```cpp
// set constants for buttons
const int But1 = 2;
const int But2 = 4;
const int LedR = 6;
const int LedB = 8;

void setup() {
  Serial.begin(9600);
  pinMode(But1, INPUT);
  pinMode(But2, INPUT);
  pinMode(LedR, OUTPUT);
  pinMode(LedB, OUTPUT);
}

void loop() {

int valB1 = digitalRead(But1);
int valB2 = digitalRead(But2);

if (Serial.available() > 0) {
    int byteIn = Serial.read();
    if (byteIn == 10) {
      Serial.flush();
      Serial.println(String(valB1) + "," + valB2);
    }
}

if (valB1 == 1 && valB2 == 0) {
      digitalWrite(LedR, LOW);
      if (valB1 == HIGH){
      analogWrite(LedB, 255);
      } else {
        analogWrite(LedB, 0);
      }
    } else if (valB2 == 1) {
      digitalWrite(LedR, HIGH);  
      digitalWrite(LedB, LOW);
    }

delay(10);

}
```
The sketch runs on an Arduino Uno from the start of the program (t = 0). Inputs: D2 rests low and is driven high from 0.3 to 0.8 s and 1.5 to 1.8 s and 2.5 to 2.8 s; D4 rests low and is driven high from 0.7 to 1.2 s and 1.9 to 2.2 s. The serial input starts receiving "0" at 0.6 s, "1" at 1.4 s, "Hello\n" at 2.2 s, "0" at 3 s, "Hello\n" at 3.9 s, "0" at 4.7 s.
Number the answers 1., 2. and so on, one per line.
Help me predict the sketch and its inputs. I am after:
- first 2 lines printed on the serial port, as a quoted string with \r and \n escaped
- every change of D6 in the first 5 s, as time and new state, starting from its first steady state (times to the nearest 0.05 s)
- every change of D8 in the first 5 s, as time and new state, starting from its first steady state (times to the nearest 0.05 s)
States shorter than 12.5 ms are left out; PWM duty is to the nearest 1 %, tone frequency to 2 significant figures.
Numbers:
1. "0,0\r\n0,0\r\n"
2. 0 s low; 0.7 s high; 1.5 s low; 1.9 s high; 2.5 s low
3. 0 s low; 0.3 s high; 0.7 s low; 1.5 s high; 1.9 s low; 2.5 s high
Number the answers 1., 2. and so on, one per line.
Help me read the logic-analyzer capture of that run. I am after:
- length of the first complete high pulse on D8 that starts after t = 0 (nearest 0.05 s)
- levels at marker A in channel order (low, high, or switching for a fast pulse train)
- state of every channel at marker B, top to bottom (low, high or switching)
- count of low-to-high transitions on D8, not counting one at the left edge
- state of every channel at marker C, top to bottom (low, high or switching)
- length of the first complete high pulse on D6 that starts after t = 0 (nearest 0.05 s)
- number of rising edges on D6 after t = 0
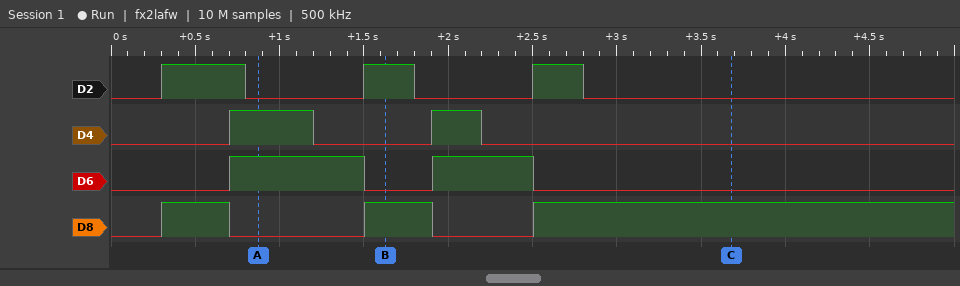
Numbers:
1. 0.40 s
2. D2 low, D4 high, D6 high, D8 low
3. D2 high, D4 low, D6 low, D8 high
4. 3
5. D2 low, D4 low, D6 low, D8 high
6. 0.80 s
7. 2
